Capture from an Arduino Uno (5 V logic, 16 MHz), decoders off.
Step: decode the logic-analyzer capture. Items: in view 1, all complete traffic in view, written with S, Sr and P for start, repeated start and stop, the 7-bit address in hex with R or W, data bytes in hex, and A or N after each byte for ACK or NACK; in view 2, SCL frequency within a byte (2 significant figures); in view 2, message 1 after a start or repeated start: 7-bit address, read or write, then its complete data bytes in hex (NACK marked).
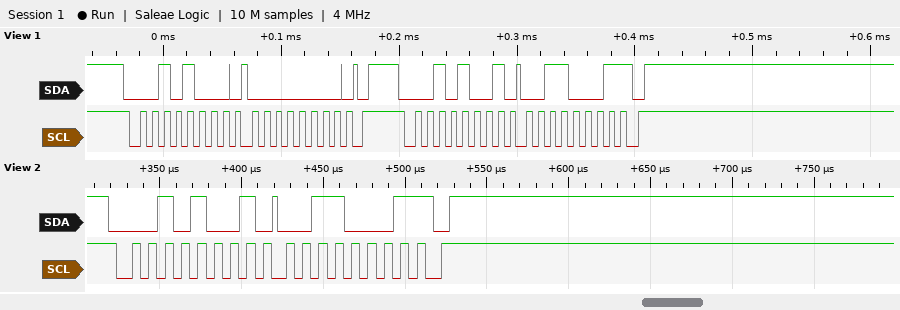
S 14W A 00 A P S 14R A 31 N P
100 kHz
0x14 read: 31 NACK
